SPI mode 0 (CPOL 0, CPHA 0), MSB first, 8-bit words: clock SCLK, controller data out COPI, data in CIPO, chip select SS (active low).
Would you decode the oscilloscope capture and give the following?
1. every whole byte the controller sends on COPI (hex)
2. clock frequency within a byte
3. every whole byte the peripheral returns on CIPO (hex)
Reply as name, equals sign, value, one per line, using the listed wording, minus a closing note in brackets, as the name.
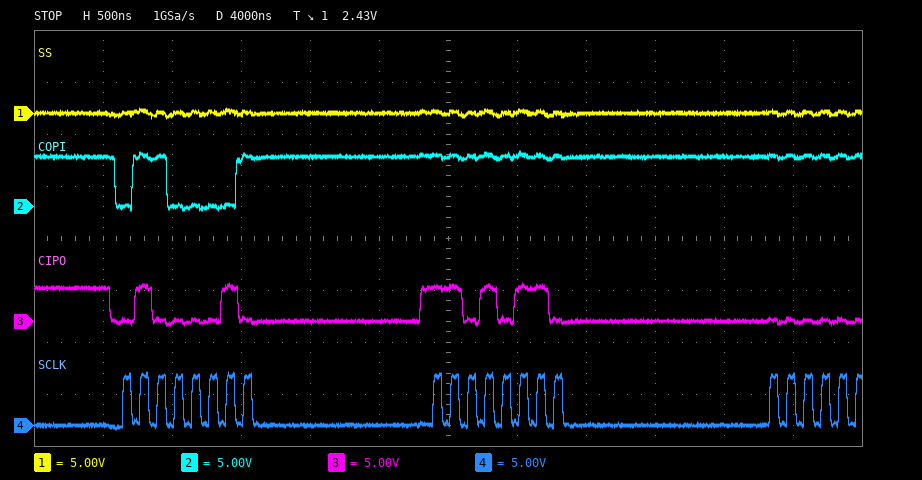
every whole byte the controller sends on COPI = 61 FF
clock frequency within a byte = 8 MHz
every whole byte the peripheral returns on CIPO = 42 D6
